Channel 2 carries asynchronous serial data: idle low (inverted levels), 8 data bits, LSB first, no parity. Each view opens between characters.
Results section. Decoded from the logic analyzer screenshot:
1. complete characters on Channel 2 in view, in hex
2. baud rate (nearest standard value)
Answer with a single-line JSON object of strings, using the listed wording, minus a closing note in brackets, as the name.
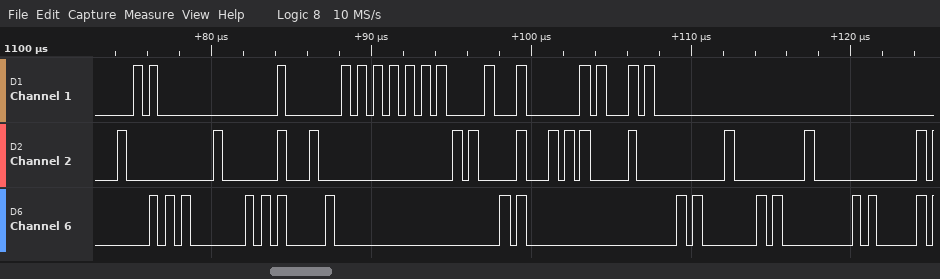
{"complete characters on Channel 2 in view, in hex": "FF, 7F, FF, 7D, F5, FF, FF, FF", "baud rate": "2000000 baud"}
